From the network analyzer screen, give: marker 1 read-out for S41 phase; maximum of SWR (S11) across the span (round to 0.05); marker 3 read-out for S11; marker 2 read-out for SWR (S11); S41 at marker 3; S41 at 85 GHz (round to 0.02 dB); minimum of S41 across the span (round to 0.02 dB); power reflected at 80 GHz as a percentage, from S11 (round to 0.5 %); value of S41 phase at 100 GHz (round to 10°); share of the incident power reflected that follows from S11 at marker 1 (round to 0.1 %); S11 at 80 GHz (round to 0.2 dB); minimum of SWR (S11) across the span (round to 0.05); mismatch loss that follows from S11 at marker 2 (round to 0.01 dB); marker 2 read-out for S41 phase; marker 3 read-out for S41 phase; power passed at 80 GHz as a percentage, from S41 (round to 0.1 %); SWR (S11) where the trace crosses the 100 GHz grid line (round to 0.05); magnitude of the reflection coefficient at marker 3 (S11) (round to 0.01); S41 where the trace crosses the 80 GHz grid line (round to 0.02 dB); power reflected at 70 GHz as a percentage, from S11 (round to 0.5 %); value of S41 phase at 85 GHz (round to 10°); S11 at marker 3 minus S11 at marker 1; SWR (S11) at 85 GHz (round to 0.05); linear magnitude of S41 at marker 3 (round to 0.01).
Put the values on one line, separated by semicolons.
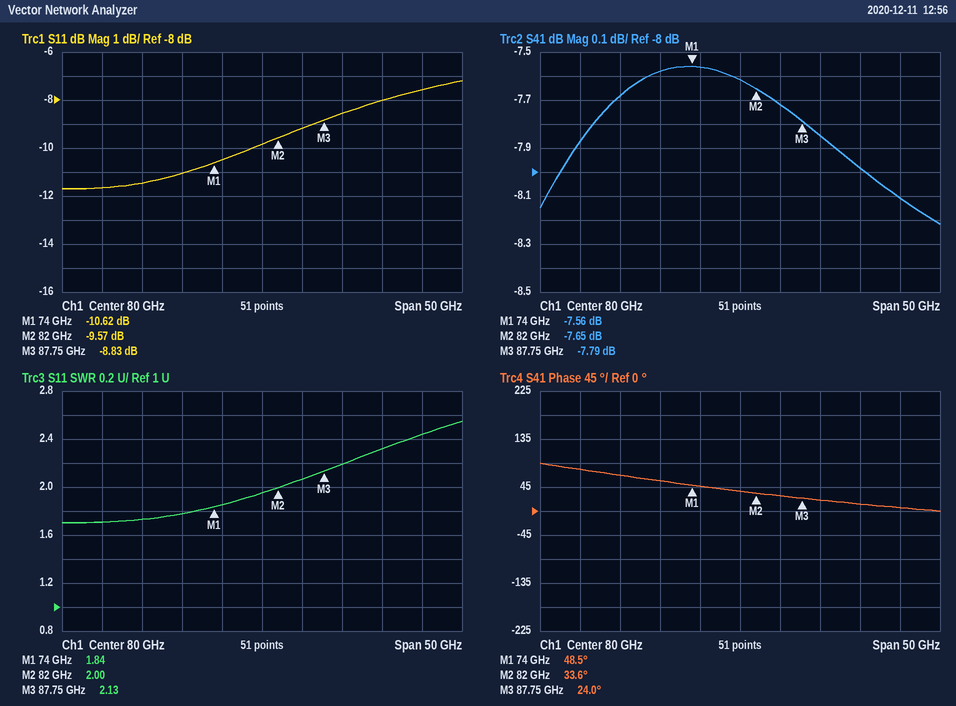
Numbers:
48.5°; 2.55; -8.83 dB; 2.00; -7.79 dB; -7.72 dB; -8.22 dB; 10.5 %; 10°; 8.7 %; -9.8 dB; 1.70; 0.51 dB; 33.6°; 24.0°; 17.3 %; 2.45; 0.36; -7.62 dB; 8.0 %; 30°; 1.79 dB; 2.05; 0.41
